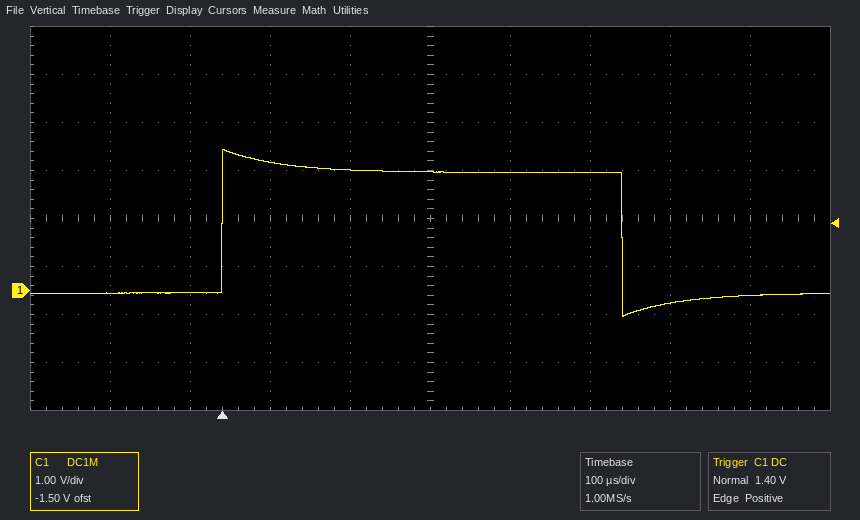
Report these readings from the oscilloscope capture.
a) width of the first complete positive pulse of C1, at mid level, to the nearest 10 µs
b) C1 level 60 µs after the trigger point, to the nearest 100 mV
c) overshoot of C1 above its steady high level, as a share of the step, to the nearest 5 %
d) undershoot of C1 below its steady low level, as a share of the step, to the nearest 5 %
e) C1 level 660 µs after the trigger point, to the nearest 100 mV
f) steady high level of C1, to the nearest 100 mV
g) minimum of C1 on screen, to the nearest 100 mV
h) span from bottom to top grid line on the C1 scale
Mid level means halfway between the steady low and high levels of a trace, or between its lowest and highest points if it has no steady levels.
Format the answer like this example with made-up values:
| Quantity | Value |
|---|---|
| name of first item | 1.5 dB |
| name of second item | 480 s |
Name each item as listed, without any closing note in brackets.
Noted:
| Quantity | Value |
|---|---|
| width of the first complete positive pulse of C1, at mid level, to the nearest 10 µs | 500 µs |
| C1 level 60 µs after the trigger point, to the nearest 100 mV | 2.7 V |
| overshoot of C1 above its steady high level, as a share of the step, to the nearest 5 % | 20 % |
| undershoot of C1 below its steady low level, as a share of the step, to the nearest 5 % | 20 % |
| C1 level 660 µs after the trigger point, to the nearest 100 mV | -100 mV |
| steady high level of C1, to the nearest 100 mV | 2.5 V |
| minimum of C1 on screen, to the nearest 100 mV | -500 mV |
| span from bottom to top grid line on the C1 scale | 8 V |
